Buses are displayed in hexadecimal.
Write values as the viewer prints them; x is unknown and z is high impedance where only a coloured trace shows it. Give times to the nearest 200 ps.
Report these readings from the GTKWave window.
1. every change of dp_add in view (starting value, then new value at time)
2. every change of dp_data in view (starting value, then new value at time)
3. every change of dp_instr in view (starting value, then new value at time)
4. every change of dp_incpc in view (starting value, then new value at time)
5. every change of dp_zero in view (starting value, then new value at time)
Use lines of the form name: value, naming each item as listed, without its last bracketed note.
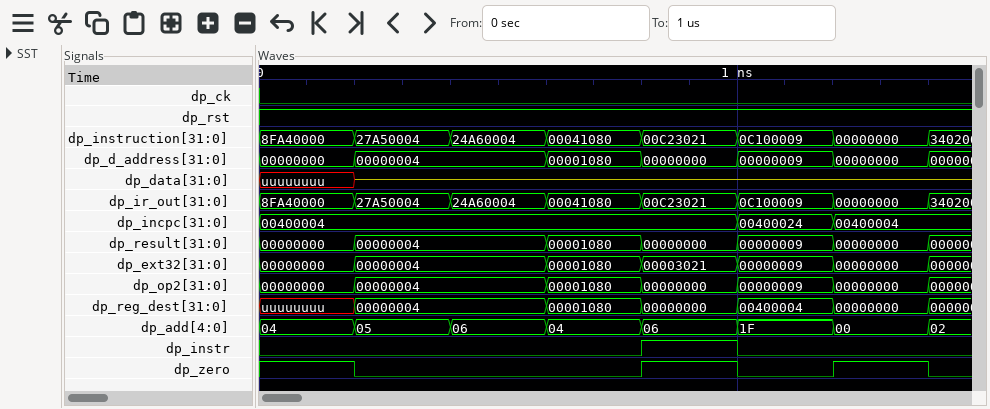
every change of dp_add in view: 04, 05 at 200 ps, 06 at 400 ps, 04 at 600 ps, 06 at 800 ps, 1F at 1000 ps, 00 at 1200 ps, 02 at 1400 ps
every change of dp_data in view: uuuuuuuu, z at 200 ps
every change of dp_instr in view: 0, 1 at 800 ps, 0 at 1000 ps
every change of dp_incpc in view: 00400004, 00400024 at 1000 ps, 00400004 at 1200 ps
every change of dp_zero in view: 1, 0 at 200 ps, 1 at 800 ps, 0 at 1000 ps, 1 at 1200 ps, 0 at 1400 ps
